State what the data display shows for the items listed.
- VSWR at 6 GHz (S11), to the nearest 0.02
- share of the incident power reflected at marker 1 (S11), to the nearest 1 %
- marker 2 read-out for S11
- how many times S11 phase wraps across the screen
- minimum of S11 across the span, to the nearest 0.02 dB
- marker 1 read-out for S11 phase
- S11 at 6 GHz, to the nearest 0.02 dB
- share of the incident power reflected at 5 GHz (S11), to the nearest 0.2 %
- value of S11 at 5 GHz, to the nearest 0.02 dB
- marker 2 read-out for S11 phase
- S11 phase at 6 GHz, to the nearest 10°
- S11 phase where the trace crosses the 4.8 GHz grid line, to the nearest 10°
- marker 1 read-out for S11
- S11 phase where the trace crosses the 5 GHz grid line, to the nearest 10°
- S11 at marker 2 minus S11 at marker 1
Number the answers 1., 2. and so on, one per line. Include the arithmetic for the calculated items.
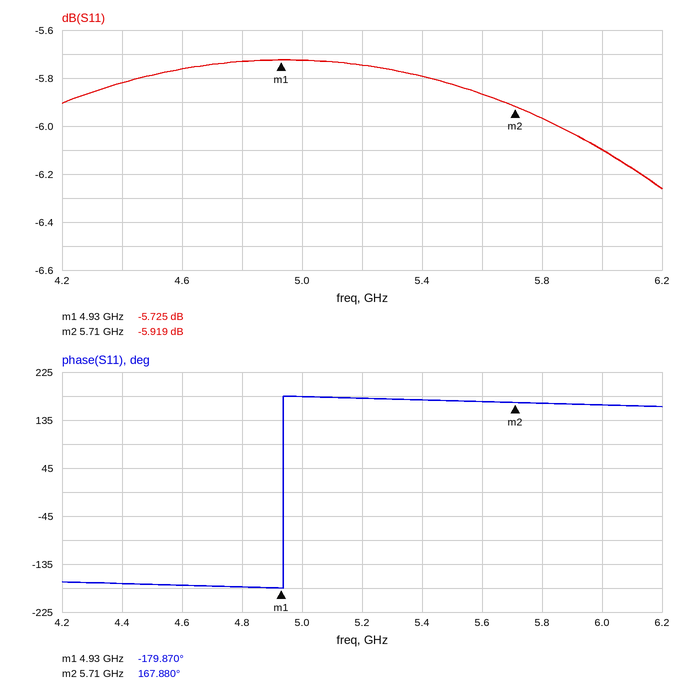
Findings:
1. |Γ| = 10^(-6.1/20) = 0.4955; VSWR = (1 + 0.4955)/(1 − 0.4955) ≈ 2.96
2. 10^(-5.725/10) ≈ 27 %
3. -5.919 dB
4. 1
5. -6.26 dB
6. -179.870°
7. -6.10 dB
8. 10^(-5.72/10) ≈ 26.8 %
9. -5.72 dB
10. 167.880°
11. 160°
12. -180°
13. -5.725 dB
14. 180°
15. -5.919 − (-5.725) = -0.194 dB
